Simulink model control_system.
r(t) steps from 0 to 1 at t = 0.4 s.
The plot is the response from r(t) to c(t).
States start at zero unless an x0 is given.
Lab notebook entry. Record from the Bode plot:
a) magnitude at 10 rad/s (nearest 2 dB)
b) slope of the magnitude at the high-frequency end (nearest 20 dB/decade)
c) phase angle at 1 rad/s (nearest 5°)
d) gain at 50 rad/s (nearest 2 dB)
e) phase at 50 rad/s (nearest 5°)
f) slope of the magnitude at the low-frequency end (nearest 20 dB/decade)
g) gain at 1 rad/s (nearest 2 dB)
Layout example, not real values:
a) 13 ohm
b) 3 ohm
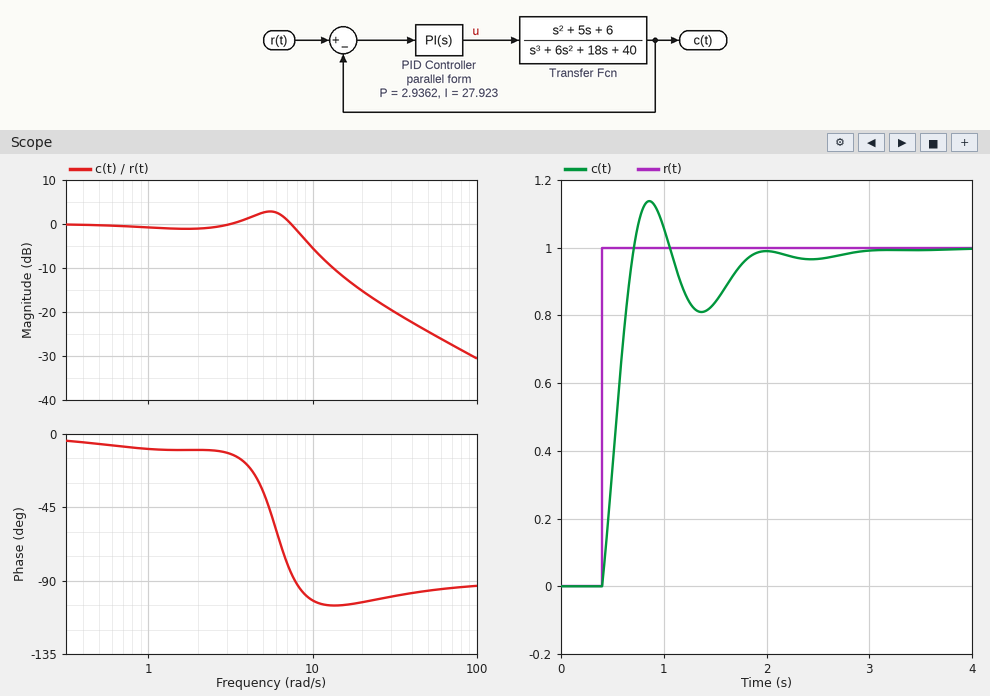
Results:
a) -6 dB
b) -20 dB/decade
c) -10°
d) -24 dB
e) -95°
f) 0 dB/decade
g) 0 dB
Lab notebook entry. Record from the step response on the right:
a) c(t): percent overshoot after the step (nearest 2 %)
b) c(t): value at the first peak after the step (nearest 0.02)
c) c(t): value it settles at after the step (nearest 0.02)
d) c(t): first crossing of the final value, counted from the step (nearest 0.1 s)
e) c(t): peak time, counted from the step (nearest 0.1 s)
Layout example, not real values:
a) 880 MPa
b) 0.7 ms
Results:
a) 14 %
b) 1.14
c) 1.00
d) 0.3 s
e) 0.5 s
